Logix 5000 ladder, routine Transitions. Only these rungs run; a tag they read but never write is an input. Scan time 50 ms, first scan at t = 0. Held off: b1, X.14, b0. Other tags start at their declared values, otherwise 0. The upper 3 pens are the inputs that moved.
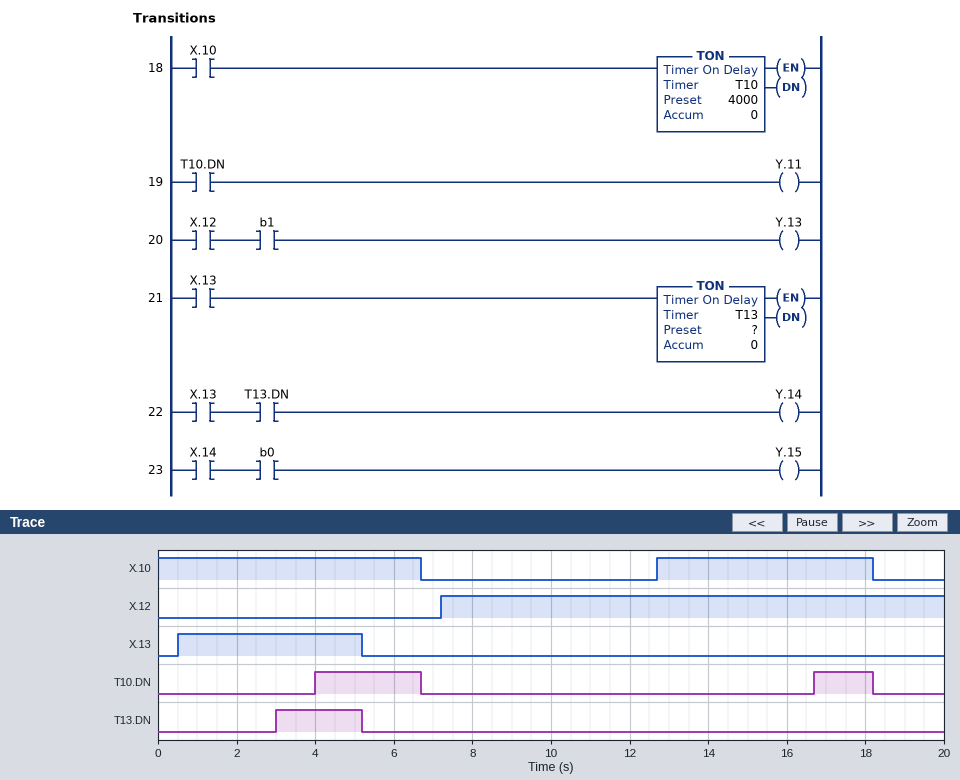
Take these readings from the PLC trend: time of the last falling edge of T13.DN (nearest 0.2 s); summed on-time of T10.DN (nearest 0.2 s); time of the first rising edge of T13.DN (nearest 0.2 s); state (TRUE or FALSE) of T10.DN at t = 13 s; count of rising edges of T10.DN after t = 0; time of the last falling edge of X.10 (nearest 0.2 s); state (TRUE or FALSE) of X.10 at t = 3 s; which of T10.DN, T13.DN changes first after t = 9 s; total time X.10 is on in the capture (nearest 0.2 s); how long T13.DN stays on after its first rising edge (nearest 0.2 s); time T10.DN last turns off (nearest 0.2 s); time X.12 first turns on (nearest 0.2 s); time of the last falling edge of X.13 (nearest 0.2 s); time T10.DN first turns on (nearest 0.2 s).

5.2 s
4.2 s
3.0 s
FALSE
2
18.2 s
TRUE
T10.DN
12.2 s
2.2 s
18.2 s
7.2 s
5.2 s
4.0 s
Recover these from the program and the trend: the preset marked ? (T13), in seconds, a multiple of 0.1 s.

2.5 s
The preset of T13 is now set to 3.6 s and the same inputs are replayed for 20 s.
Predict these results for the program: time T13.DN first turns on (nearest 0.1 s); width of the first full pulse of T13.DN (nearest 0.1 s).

4.1 s
1.1 s
